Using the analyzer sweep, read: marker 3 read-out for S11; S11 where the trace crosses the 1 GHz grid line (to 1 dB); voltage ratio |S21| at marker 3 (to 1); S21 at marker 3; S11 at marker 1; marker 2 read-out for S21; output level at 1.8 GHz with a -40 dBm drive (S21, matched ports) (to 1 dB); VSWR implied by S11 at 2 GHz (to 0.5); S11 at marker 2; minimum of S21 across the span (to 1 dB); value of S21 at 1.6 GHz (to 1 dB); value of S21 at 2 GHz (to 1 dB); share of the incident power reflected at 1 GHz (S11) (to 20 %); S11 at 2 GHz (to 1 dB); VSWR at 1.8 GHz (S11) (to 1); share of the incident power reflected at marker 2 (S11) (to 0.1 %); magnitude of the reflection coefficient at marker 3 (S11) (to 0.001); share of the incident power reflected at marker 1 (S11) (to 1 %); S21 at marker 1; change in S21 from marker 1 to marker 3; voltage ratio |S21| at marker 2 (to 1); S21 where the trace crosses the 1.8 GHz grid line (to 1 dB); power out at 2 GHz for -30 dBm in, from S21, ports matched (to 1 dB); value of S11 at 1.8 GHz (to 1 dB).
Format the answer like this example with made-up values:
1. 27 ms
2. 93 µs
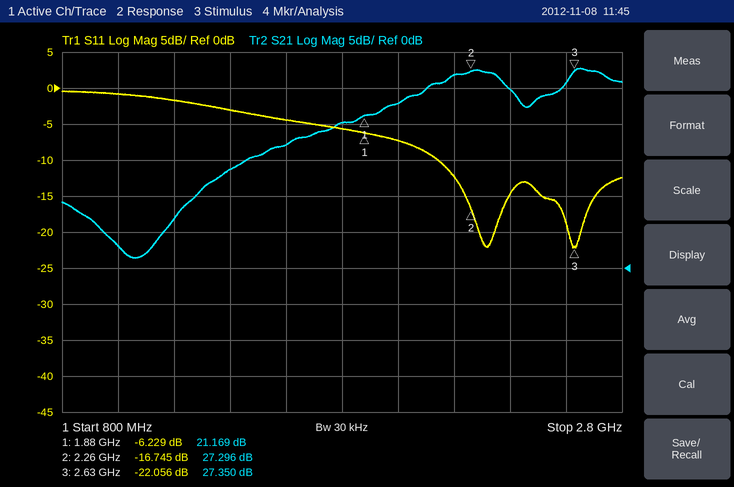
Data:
1. -22.056 dB
2. -1 dB
3. 23
4. 27.350 dB
5. -6.229 dB
6. 27.296 dB
7. -20 dBm
8. 2.5
9. -16.745 dB
10. 1 dB
11. 17 dB
12. 23 dB
13. 80 %
14. -7 dB
15. 3
16. 2.1 %
17. 0.079
18. 24 %
19. 21.169 dB
20. 6.181 dB
21. 23
22. 20 dB
23. -7 dBm
24. -6 dB
